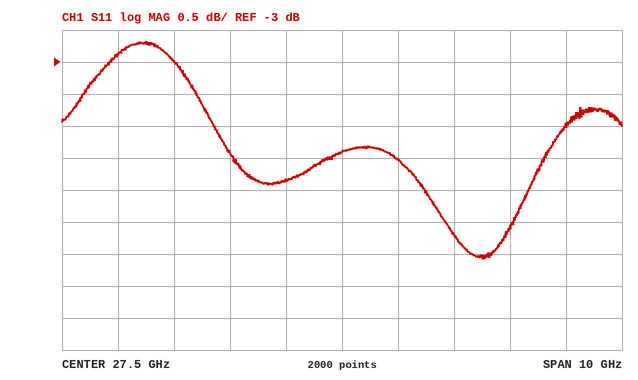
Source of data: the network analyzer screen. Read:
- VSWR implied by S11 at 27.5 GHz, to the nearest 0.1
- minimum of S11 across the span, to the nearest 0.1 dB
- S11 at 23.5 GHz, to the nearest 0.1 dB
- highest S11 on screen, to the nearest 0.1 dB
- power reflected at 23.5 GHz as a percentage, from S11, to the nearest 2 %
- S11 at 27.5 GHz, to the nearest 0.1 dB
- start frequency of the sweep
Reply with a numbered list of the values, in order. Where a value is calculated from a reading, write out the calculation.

1. |Γ| = 10^(-4.4/20) = 0.6026; VSWR = (1 + 0.6026)/(1 − 0.6026) ≈ 4.0
2. -6.1 dB
3. -2.9 dB
4. -2.7 dB
5. 10^(-2.9/10) ≈ 51.3 %, so 52 % to the nearest 2 %
6. -4.4 dB
7. 22.5 GHz
